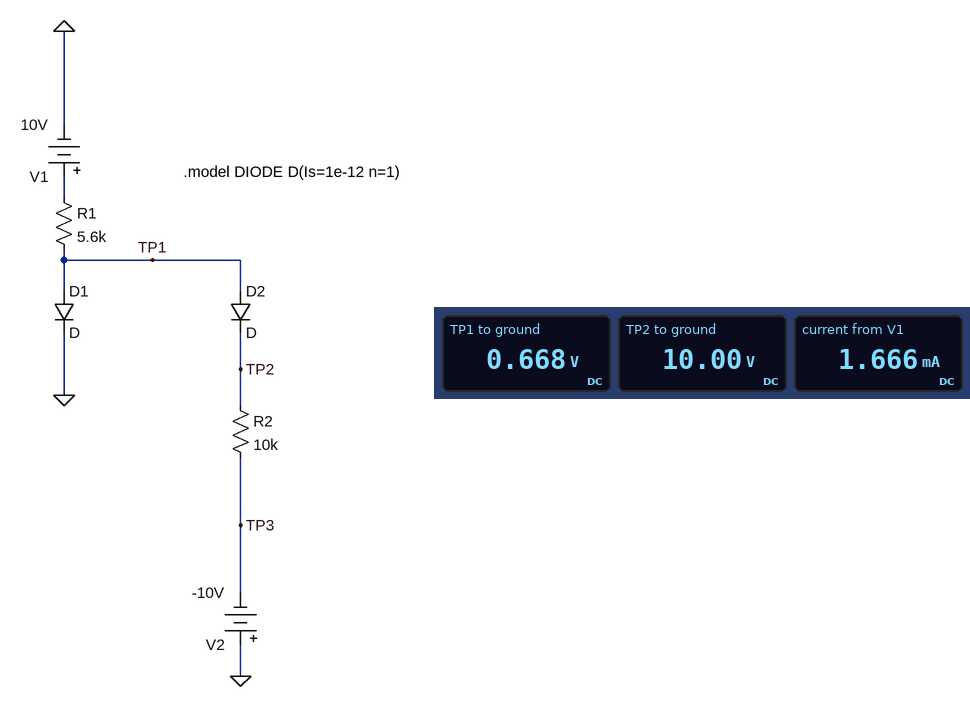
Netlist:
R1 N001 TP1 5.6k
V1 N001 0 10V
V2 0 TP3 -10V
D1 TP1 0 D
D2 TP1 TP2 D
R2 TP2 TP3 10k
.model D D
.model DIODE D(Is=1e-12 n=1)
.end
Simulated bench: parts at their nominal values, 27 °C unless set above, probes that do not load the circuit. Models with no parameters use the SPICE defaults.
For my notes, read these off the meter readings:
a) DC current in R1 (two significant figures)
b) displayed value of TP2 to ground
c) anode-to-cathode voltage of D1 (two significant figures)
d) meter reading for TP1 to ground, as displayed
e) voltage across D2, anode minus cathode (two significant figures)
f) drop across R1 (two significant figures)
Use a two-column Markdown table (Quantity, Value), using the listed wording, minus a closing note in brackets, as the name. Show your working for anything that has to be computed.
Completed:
| Quantity | Value |
|---|---|
| DC current in R1 | (10 V - 668 mV) / 5.6 kΩ = 1.7 mA |
| displayed value of TP2 to ground | 10.00 V |
| anode-to-cathode voltage of D1 | 668 mV = 670 mV |
| meter reading for TP1 to ground, as displayed | 0.668 V |
| voltage across D2, anode minus cathode | 668 mV - 10 V = -9.3 V |
| drop across R1 | 10 V - 668 mV = 9.3 V |
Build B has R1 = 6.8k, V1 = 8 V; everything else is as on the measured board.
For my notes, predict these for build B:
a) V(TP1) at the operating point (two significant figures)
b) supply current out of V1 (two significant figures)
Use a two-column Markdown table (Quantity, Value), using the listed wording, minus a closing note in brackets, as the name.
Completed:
| Quantity | Value |
|---|---|
| V(TP1) at the operating point | 660 mV |
| supply current out of V1 | 1.1 mA |
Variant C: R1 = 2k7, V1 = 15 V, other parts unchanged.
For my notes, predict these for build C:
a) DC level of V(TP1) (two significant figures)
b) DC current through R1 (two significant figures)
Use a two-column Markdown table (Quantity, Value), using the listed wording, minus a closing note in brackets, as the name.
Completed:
| Quantity | Value |
|---|---|
| DC level of V(TP1) | 700 mV |
| DC current through R1 | 5.3 mA |
